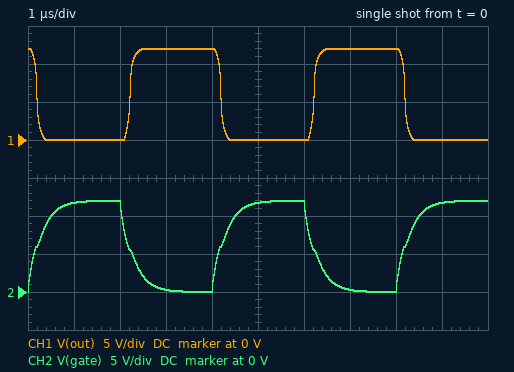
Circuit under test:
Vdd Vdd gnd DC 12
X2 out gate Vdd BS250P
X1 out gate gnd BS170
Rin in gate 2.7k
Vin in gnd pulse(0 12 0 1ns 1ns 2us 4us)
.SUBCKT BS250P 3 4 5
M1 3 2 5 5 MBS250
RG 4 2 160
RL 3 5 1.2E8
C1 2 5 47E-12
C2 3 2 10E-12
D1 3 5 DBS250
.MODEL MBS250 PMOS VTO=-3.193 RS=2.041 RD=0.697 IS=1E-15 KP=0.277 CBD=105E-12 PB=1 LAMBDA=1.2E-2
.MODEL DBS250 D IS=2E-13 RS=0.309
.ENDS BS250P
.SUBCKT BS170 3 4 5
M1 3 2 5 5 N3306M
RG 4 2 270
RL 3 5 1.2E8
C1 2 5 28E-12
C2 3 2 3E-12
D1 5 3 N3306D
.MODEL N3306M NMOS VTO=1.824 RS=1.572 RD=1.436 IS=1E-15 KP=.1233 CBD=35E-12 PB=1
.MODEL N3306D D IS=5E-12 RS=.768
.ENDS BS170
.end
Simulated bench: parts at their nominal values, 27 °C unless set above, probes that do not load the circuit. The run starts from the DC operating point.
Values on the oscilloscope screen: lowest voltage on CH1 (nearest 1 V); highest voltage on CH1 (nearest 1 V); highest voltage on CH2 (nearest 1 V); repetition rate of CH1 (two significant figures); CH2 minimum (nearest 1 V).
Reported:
0 V
12 V
12 V
250 kHz
0 V
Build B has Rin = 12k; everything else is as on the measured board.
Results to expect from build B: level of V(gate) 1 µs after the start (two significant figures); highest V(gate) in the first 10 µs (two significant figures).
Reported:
6.2 V
10 V
